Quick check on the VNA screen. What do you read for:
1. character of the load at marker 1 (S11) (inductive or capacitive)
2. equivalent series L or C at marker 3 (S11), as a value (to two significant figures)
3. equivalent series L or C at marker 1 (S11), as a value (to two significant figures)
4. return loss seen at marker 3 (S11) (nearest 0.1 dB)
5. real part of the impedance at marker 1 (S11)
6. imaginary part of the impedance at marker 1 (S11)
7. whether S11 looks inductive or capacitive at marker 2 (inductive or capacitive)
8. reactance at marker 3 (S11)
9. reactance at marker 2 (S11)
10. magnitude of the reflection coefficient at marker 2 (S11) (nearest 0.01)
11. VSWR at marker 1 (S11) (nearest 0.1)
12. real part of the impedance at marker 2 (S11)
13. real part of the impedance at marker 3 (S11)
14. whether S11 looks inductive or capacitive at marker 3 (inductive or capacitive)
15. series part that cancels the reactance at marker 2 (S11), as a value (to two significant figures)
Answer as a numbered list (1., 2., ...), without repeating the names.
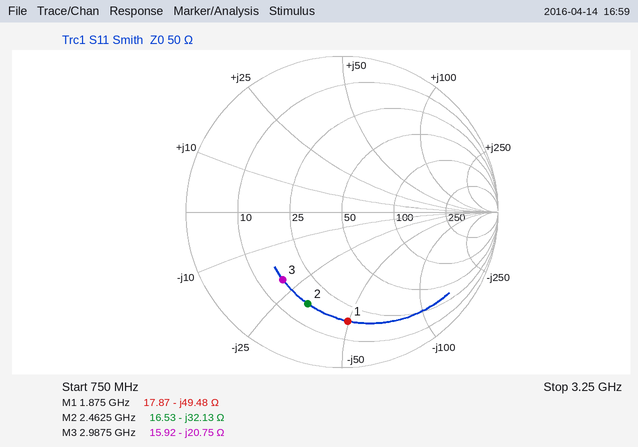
1. capacitive
2. 2.6 pF
3. 1.7 pF
4. 4.8 dB
5. 17.87 Ω
6. -49.48 Ω
7. capacitive
8. -20.75 Ω
9. -32.13 Ω
10. 0.63
11. 5.7
12. 16.53 Ω
13. 15.92 Ω
14. capacitive
15. 2.1 nH
